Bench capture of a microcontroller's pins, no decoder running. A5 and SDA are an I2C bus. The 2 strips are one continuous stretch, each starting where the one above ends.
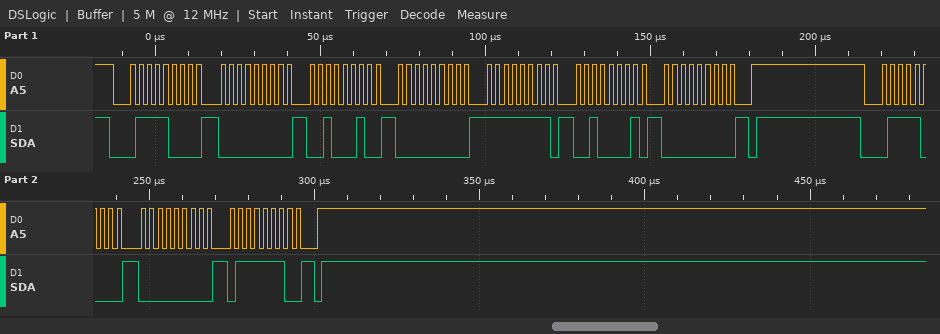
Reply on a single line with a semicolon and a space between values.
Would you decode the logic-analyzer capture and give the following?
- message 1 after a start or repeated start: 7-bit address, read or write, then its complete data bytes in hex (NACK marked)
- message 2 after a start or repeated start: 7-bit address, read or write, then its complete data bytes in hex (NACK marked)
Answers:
0x3C write: 00 22 00 FF 21 00; 0x3C write: 00 7E
